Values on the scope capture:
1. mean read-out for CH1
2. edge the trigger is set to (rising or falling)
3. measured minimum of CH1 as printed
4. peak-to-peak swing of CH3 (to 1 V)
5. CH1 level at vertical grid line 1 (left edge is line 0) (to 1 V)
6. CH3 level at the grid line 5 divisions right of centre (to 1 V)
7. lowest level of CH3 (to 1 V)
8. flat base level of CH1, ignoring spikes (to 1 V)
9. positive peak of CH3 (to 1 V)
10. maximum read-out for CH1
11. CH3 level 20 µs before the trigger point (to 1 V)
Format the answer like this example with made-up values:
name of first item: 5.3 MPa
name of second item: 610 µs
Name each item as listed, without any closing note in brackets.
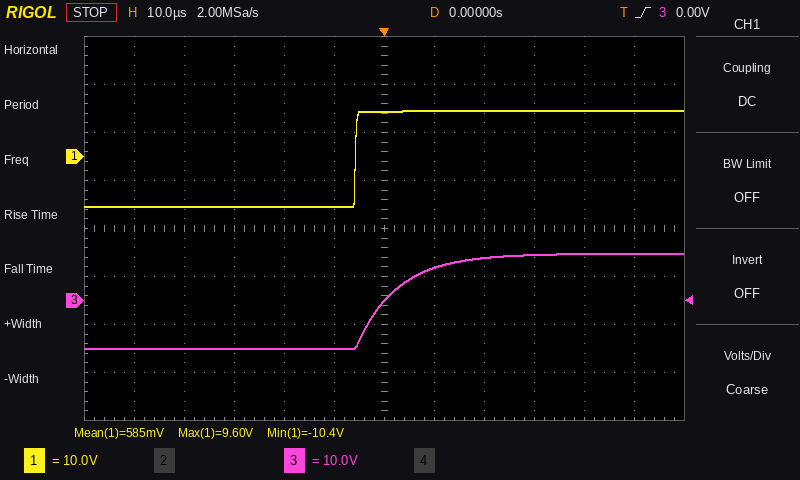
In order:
mean read-out for CH1: 585 mV
edge the trigger is set to: rising
measured minimum of CH1 as printed: -10.4 V
peak-to-peak swing of CH3: 20 V
CH1 level at vertical grid line 1 (left edge is line 0): -10 V
CH3 level at the grid line 5 divisions right of centre: 10 V
lowest level of CH3: -10 V
flat base level of CH1, ignoring spikes: -10 V
positive peak of CH3: 10 V
maximum read-out for CH1: 9.60 V
CH3 level 20 µs before the trigger point: -10 V
